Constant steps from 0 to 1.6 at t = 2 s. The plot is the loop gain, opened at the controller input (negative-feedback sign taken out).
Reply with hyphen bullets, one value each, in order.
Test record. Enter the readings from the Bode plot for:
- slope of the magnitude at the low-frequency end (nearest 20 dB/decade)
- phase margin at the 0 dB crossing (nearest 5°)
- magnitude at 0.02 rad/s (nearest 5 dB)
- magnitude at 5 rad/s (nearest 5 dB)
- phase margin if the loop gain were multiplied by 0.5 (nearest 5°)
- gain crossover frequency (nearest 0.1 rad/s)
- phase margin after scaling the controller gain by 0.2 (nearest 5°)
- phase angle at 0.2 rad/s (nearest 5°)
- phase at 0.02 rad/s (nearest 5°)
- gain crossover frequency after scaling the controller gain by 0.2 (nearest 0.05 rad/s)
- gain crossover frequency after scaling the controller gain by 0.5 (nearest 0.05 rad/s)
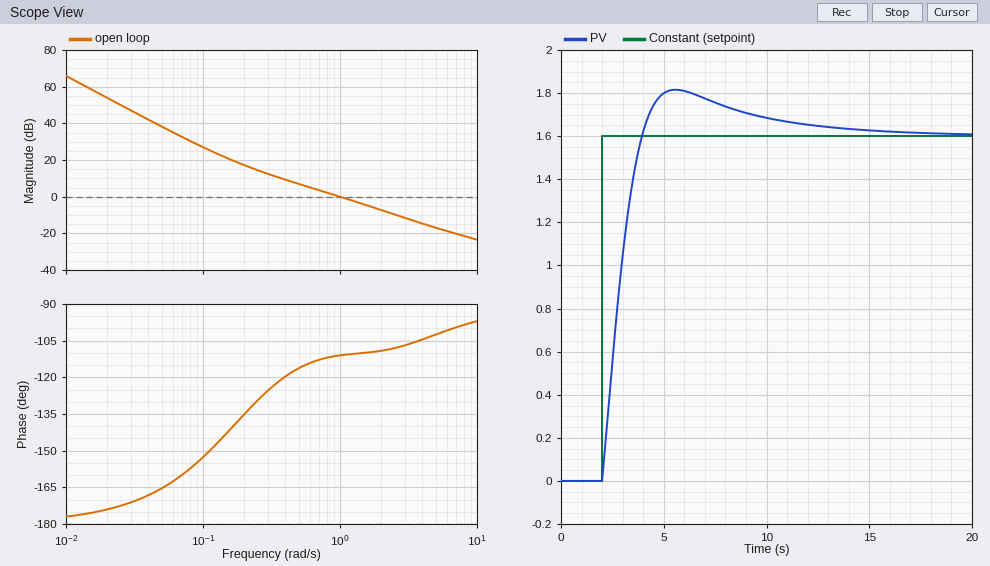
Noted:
- -40 dB/decade
- 70°
- 55 dB
- -15 dB
- 65°
- 1.0 rad/s
- 50°
- -135°
- -175°
- 0.25 rad/s
- 0.55 rad/s
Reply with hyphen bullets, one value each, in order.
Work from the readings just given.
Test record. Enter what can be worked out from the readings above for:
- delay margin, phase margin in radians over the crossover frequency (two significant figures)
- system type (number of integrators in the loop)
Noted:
- 1.2 s
- 2
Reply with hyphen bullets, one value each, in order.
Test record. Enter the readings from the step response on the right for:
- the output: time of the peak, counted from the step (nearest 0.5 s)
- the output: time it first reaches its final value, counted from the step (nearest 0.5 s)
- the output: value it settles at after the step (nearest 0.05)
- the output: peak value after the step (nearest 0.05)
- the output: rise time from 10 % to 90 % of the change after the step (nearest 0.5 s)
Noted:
- 3.5 s
- 2.0 s
- 1.60
- 1.80
- 1.5 s
